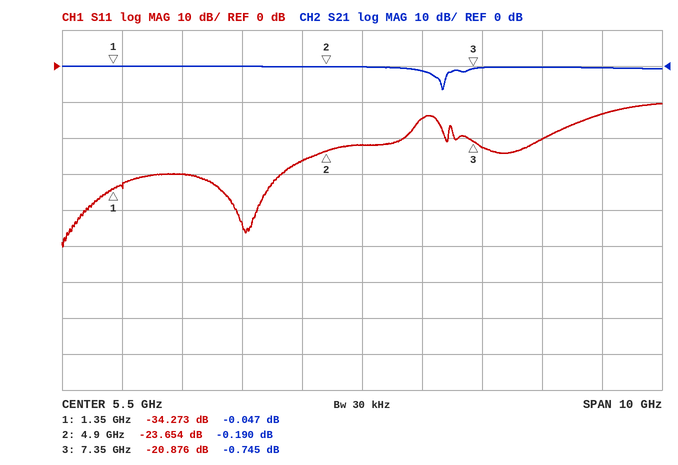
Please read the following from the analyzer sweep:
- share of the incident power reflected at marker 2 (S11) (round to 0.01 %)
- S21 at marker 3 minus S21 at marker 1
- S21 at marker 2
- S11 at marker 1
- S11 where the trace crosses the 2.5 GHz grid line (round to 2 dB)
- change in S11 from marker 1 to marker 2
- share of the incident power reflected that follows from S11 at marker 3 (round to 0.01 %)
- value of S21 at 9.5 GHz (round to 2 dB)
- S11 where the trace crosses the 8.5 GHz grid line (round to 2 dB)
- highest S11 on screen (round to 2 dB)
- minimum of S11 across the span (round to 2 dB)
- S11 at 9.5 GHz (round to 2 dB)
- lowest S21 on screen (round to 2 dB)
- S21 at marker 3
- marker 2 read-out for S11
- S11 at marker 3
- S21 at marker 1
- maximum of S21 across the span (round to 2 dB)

0.43 %
-0.698 dB
-0.190 dB
-34.273 dB
-30 dB
10.619 dB
0.82 %
0 dB
-20 dB
-10 dB
-50 dB
-14 dB
-6 dB
-0.745 dB
-23.654 dB
-20.876 dB
-0.047 dB
0 dB
